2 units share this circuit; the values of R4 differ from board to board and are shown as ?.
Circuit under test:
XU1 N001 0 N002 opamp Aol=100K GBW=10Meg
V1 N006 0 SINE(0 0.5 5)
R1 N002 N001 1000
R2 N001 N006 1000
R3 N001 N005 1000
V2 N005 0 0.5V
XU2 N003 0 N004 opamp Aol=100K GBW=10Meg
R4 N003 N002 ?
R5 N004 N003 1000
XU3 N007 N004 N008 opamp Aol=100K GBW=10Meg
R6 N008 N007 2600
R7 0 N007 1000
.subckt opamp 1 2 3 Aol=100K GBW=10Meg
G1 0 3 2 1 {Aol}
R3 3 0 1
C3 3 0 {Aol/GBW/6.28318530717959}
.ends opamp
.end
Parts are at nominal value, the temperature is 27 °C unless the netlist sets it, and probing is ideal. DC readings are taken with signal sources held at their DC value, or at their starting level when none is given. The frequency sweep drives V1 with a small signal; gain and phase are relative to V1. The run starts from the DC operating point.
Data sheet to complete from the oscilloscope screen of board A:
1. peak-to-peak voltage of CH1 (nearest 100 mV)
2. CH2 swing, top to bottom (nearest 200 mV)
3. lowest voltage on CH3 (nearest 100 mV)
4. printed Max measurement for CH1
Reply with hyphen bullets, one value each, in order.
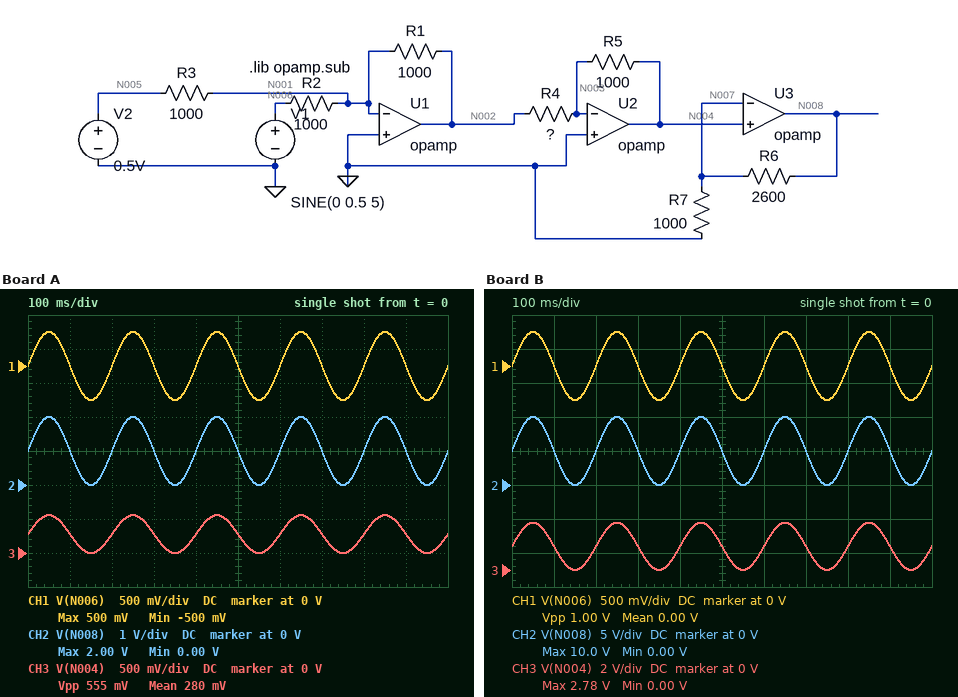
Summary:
- 1.0 V
- 2.0 V
- 0 V
- 500 mV
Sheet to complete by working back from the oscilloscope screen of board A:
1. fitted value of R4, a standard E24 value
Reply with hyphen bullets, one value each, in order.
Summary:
- 1.8 kΩ
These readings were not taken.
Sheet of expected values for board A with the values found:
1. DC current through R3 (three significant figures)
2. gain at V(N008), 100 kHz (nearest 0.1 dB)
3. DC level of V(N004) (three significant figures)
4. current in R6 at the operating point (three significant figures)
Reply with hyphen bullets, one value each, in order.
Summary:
- 500 µA
- 6.0 dB
- 278 mV
- 278 µA
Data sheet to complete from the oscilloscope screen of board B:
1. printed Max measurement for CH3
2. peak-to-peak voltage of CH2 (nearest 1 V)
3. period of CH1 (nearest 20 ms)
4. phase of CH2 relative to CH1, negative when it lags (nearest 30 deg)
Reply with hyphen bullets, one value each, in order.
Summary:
- 2.78 V
- 10 V
- 200 ms
- 0 deg
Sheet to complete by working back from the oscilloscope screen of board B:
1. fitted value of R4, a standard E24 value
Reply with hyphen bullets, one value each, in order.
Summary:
- 360 Ω
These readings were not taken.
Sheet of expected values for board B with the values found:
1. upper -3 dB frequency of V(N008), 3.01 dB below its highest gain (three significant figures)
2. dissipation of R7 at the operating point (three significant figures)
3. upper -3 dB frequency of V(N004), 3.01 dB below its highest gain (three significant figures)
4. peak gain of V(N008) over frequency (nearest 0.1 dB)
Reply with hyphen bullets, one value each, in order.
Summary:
- 1.47 MHz
- 1.93 mW
- 1.89 MHz
- 20.0 dB
